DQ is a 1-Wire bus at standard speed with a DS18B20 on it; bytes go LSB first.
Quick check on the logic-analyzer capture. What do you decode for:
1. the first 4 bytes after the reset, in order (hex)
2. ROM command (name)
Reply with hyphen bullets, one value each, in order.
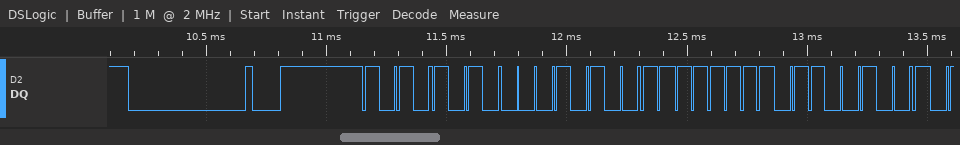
- 55 28 FF 26
- Match ROM
